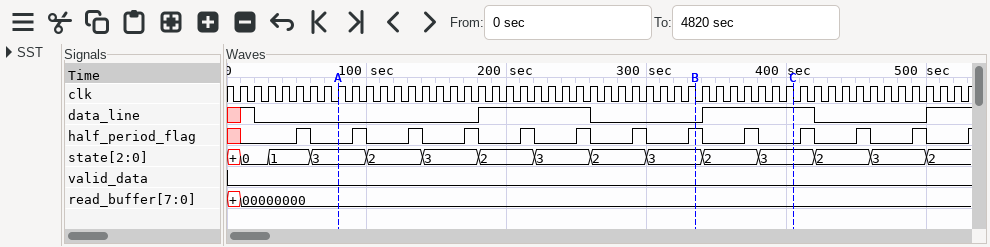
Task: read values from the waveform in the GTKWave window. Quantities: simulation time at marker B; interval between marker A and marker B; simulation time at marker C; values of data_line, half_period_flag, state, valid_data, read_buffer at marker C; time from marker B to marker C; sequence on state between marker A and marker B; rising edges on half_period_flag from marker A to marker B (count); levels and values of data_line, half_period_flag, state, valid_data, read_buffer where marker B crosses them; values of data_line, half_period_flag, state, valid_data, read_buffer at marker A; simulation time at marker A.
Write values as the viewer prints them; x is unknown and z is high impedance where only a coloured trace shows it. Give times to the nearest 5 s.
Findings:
335 s
255 s
405 s
data_line=1, half_period_flag=0, state=3, valid_data=0, read_buffer=00000000
70 s
3, 2, 3, 2, 3, 2, 3
7
data_line=0, half_period_flag=1, state=3, valid_data=0, read_buffer=00000000
data_line=0, half_period_flag=0, state=3, valid_data=0, read_buffer=00000000
80 s
